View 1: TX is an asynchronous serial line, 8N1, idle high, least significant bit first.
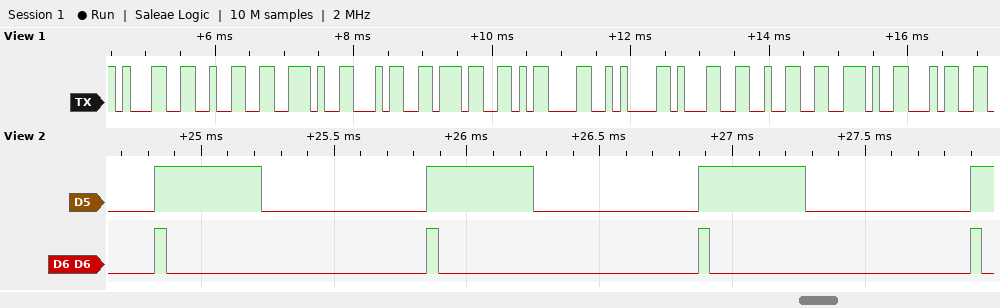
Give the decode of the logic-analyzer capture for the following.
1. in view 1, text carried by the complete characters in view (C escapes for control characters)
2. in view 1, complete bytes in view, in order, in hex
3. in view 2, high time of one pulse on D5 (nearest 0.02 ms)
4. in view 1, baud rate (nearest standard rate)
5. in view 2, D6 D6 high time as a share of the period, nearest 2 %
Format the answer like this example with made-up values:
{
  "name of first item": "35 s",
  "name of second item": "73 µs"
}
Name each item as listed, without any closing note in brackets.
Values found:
{
  "in view 1, text carried by the complete characters in view": "\"12.47\\r\\n12.4\"",
  "in view 1, complete bytes in view, in order, in hex": "31 32 2E 34 37 0D 0A 31 32 2E 34",
  "in view 2, high time of one pulse on D5": "0.40 ms",
  "in view 1, baud rate": "9600 baud",
  "in view 2, D6 D6 high time as a share of the period, nearest 2 %": "4 %"
}
